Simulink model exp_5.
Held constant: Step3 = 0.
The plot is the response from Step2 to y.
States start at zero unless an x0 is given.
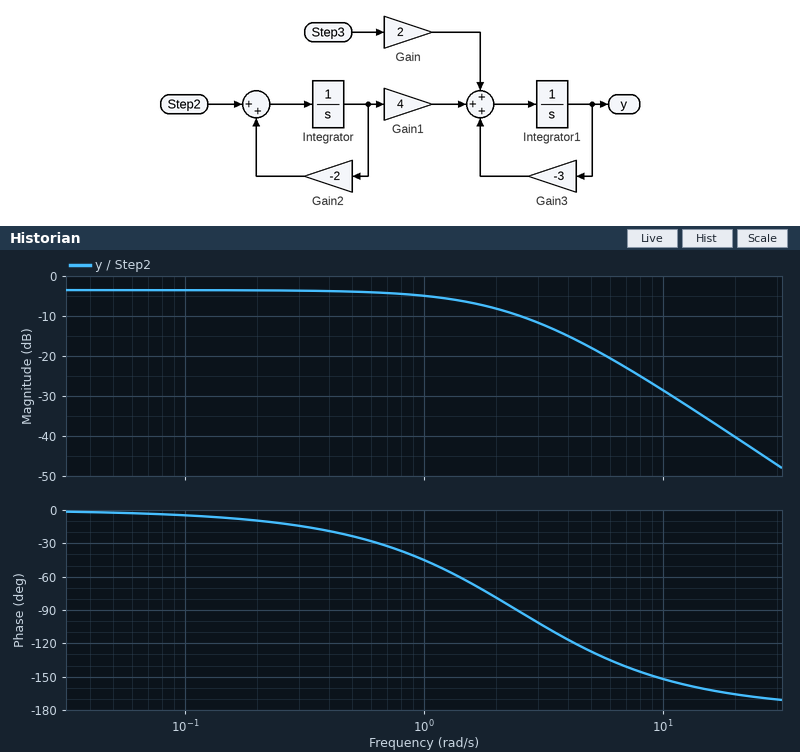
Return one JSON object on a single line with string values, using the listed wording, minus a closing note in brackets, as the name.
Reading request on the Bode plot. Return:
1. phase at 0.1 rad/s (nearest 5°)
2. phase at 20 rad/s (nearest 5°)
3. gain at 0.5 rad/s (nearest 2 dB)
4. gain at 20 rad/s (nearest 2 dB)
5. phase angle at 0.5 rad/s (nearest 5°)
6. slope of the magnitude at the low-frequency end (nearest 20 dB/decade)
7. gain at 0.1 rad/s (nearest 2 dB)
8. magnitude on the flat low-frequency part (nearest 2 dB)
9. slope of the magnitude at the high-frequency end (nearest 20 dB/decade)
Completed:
{"phase at 0.1 rad/s": "-5°", "phase at 20 rad/s": "-165°", "gain at 0.5 rad/s": "-4 dB", "gain at 20 rad/s": "-40 dB", "phase angle at 0.5 rad/s": "-25°", "slope of the magnitude at the low-frequency end": "0 dB/decade", "gain at 0.1 rad/s": "-4 dB", "magnitude on the flat low-frequency part": "-4 dB", "slope of the magnitude at the high-frequency end": "-40 dB/decade"}
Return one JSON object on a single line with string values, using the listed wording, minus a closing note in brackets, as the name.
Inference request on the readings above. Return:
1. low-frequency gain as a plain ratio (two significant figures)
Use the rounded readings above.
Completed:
{"low-frequency gain as a plain ratio": "0.63"}
